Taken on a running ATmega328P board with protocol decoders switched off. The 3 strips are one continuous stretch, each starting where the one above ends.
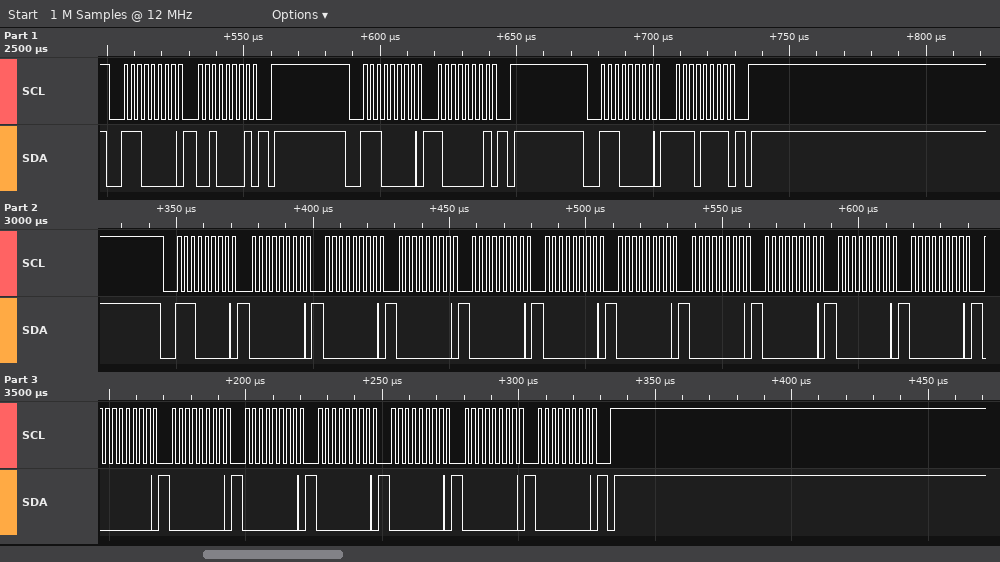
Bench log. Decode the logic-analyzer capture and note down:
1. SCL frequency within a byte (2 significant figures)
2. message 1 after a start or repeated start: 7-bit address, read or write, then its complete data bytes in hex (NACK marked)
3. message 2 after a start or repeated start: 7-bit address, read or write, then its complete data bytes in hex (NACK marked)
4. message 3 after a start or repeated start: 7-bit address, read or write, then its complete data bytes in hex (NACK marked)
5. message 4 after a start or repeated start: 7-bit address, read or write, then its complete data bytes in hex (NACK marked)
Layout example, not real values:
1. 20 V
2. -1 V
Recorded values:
1. 400 kHz
2. 0x70 write: 21
3. 0x70 write: 81
4. 0x70 write: EF
5. 0x70 write: 00 00 00 00 00 00 00 00 00 00 00 00 00 00 00 00 00
